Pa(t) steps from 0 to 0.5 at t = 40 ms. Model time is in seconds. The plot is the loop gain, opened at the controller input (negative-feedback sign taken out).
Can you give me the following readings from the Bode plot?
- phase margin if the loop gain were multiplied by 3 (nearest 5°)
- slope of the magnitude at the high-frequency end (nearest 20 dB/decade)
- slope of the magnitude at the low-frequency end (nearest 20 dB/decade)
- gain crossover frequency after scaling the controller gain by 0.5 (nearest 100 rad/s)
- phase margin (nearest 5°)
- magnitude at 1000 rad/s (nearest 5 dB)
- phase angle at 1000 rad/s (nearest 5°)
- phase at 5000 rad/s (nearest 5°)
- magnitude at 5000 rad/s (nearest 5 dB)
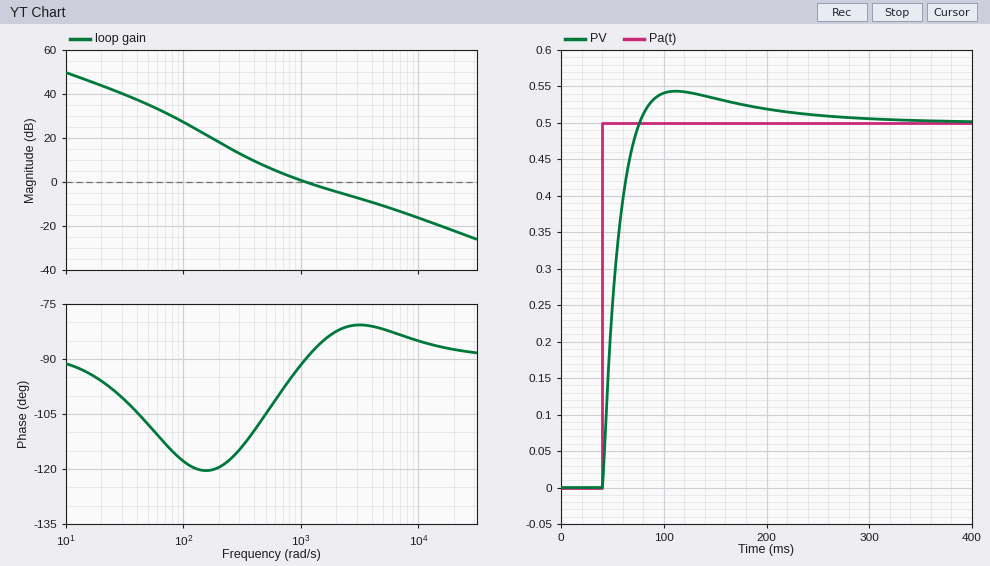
100°
-20 dB/decade
-20 dB/decade
600 rad/s
90°
0 dB
-90°
-80°
-10 dB
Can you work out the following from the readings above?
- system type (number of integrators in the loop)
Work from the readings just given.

1
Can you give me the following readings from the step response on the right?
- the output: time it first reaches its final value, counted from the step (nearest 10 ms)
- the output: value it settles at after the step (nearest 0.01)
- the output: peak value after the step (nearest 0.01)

40 ms
0.50
0.54
